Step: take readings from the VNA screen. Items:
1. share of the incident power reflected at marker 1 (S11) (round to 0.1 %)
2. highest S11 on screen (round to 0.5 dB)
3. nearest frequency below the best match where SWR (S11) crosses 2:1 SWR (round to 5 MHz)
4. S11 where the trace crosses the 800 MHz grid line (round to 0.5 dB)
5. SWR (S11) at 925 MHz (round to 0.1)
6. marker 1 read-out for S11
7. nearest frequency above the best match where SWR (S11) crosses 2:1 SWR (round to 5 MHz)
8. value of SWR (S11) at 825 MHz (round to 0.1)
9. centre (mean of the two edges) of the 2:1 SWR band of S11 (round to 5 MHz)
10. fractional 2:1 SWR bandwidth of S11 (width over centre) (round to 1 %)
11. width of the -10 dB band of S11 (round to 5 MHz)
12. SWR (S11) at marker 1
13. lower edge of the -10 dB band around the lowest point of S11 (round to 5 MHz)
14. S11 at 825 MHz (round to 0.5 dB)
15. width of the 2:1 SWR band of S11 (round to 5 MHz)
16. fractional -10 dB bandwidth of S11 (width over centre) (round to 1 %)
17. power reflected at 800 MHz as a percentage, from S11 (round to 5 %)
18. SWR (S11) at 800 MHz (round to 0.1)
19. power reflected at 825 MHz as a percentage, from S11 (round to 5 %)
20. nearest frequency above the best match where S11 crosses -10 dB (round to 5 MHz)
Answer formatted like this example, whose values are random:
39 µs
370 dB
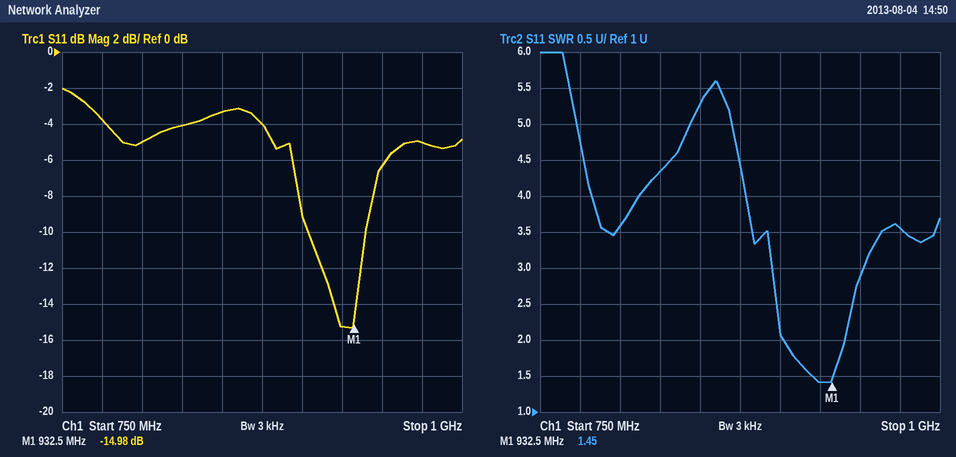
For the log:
3.2 %
-2.0 dB
900 MHz
-5.0 dB
1.4
-14.98 dB
940 MHz
4.3
920 MHz
4 %
35 MHz
1.45
905 MHz
-4.0 dB
40 MHz
4 %
30 %
3.6
40 %
940 MHz
